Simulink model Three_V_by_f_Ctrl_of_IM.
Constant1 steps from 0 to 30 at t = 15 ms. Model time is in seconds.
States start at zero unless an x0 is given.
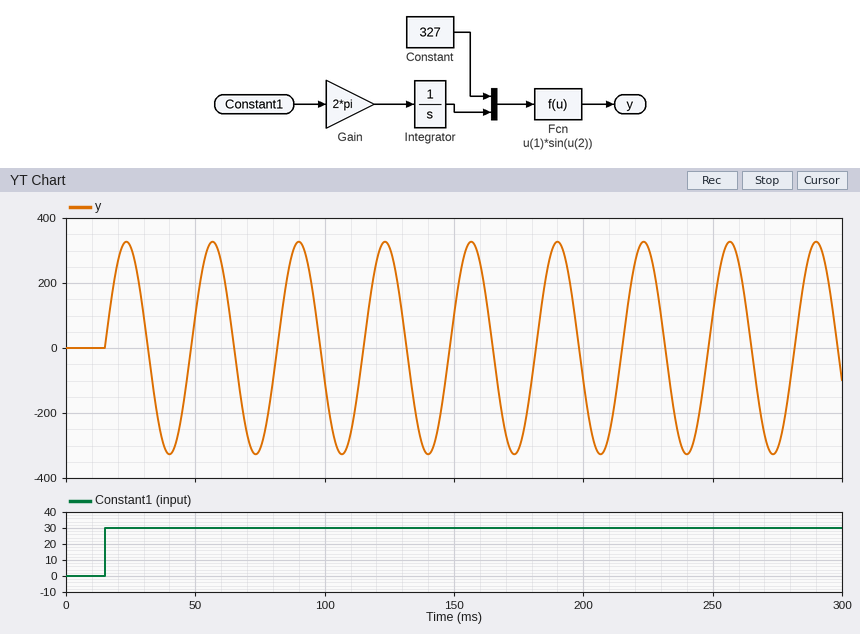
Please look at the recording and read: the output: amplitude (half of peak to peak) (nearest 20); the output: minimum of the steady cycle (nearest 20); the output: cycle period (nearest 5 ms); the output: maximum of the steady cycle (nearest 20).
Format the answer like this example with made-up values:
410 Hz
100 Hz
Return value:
320
-320
35 ms
320
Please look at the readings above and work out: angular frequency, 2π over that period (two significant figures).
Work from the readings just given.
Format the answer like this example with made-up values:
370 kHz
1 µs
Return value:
0.18 rad/ms
